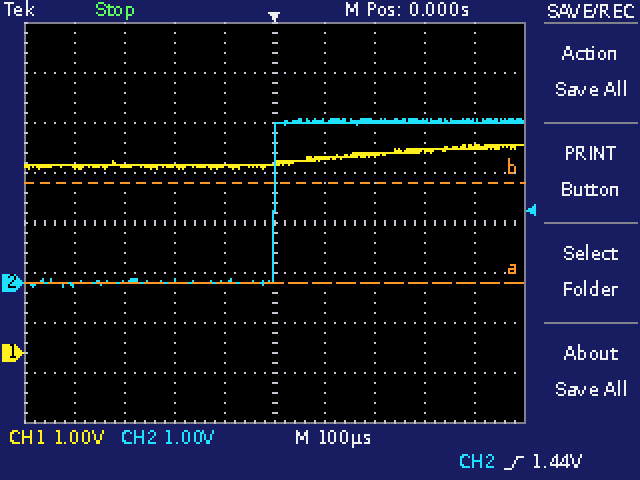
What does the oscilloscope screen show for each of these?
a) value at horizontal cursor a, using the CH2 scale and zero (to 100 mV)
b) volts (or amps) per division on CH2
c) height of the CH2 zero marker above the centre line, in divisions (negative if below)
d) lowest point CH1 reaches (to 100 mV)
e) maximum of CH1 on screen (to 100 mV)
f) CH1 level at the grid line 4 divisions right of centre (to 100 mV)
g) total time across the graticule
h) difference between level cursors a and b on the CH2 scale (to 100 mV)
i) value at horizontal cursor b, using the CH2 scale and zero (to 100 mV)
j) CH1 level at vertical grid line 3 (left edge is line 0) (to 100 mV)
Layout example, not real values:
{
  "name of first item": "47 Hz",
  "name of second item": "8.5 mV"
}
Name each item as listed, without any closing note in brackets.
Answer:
{
  "value at horizontal cursor a, using the CH2 scale and zero": "0.0 V",
  "volts (or amps) per division on CH2": "1 V",
  "height of the CH2 zero marker above the centre line, in divisions": "-1.2 div",
  "lowest point CH1 reaches": "3.7 V",
  "maximum of CH1 on screen": "4.2 V",
  "CH1 level at the grid line 4 divisions right of centre": "4.1 V",
  "total time across the graticule": "1 ms",
  "difference between level cursors a and b on the CH2 scale": "2.0 V",
  "value at horizontal cursor b, using the CH2 scale and zero": "2.0 V",
  "CH1 level at vertical grid line 3 (left edge is line 0)": "3.7 V"
}
